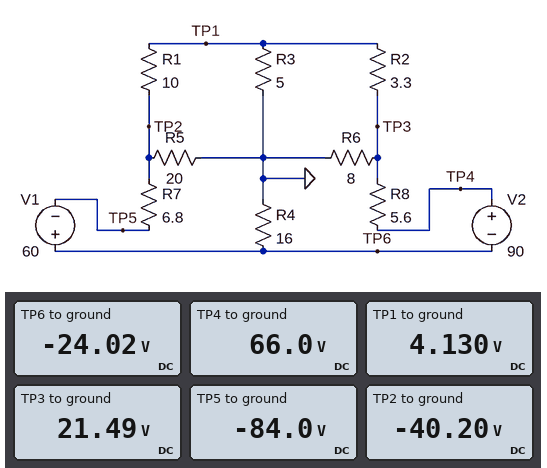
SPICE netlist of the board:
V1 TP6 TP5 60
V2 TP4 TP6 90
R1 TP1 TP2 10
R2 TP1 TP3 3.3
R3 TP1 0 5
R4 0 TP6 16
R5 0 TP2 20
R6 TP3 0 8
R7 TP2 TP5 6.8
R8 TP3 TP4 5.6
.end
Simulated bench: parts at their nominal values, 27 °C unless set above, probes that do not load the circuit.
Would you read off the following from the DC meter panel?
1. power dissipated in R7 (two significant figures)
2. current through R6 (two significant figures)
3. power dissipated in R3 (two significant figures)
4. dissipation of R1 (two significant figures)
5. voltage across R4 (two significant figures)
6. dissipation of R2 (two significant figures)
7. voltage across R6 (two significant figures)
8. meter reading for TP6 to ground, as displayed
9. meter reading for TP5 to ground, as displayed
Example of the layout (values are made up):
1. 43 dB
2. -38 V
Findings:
1. 280 W
2. 2.7 A
3. 3.4 W
4. 200 W
5. 24 V
6. 91 W
7. 21 V
8. -24.02 V
9. -84.0 V
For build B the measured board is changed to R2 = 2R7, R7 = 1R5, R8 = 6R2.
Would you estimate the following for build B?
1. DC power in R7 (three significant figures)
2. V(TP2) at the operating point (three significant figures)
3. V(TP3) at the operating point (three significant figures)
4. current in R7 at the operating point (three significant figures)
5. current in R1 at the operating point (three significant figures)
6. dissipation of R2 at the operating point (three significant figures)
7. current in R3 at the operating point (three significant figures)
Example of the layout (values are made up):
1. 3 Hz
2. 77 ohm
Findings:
1. 117 W
2. -56.5 V
3. 21.7 V
4. 8.83 A
5. 6.01 A
6. 122 W
7. 716 mA
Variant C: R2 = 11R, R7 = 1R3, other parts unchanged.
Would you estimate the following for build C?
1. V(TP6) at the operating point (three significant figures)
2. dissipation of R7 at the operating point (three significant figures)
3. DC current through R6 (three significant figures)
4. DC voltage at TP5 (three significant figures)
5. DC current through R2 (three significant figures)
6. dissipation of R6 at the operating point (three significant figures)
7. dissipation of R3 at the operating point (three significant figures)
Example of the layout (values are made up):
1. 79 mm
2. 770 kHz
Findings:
1. -7.11 V
2. 81.3 W
3. 4.51 A
4. -67.1 V
5. 3.84 A
6. 163 W
7. 7.54 W
